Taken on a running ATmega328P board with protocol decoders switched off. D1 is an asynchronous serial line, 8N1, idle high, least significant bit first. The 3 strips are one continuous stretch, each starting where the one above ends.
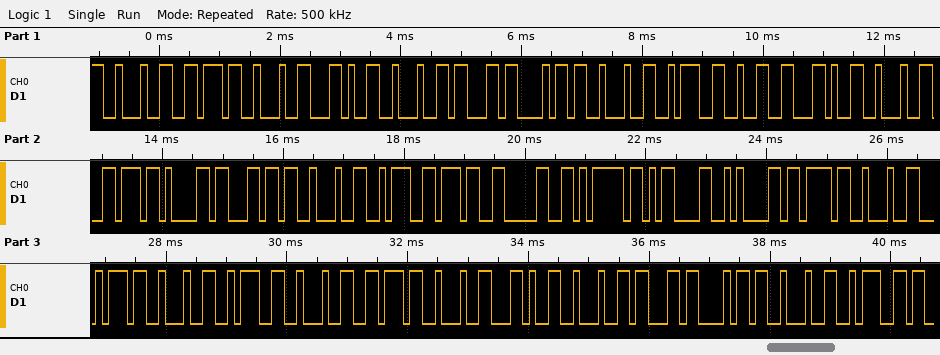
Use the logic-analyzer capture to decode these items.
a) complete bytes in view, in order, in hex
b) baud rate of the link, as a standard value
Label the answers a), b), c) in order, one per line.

a) 22 76 22 2C 22 63 68 22 3A 32 2C 22 76 61 6C 22 3A 37 30 7D 0D 0A 7B 22 74 22 3A 22 76 22 2C 22 63 68 22 3A
b) 9600 baud
